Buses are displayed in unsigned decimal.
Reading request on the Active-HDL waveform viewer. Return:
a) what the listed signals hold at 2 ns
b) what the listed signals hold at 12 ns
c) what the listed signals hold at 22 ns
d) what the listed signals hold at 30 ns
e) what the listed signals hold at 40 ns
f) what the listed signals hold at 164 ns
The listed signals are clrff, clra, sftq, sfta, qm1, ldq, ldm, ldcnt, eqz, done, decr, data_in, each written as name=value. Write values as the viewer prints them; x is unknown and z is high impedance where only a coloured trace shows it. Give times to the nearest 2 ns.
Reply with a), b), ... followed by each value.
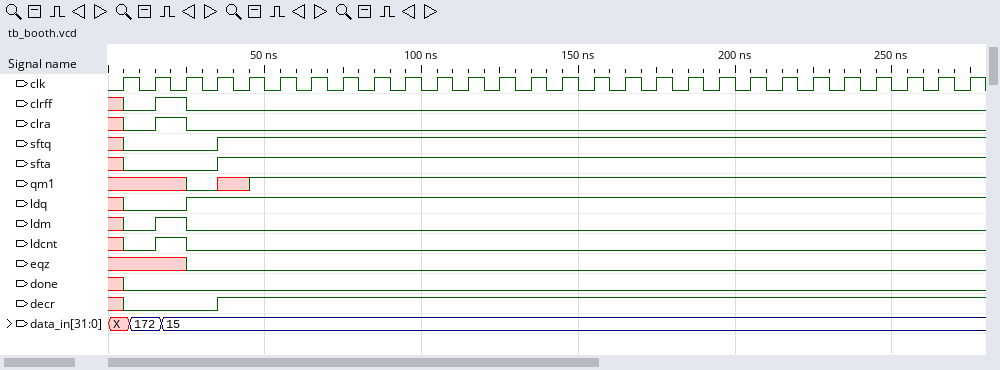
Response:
a) clrff=x, clra=x, sftq=x, sfta=x, qm1=x, ldq=x, ldm=x, ldcnt=x, eqz=x, done=x, decr=x, data_in=X
b) clrff=0, clra=0, sftq=0, sfta=0, qm1=x, ldq=0, ldm=0, ldcnt=0, eqz=x, done=0, decr=0, data_in=172
c) clrff=1, clra=1, sftq=0, sfta=0, qm1=x, ldq=0, ldm=1, ldcnt=1, eqz=x, done=0, decr=0, data_in=15
d) clrff=0, clra=0, sftq=0, sfta=0, qm1=0, ldq=1, ldm=0, ldcnt=0, eqz=0, done=0, decr=0, data_in=15
e) clrff=0, clra=0, sftq=1, sfta=1, qm1=x, ldq=1, ldm=0, ldcnt=0, eqz=0, done=0, decr=1, data_in=15
f) clrff=0, clra=0, sftq=1, sfta=1, qm1=1, ldq=1, ldm=0, ldcnt=0, eqz=0, done=0, decr=1, data_in=15
